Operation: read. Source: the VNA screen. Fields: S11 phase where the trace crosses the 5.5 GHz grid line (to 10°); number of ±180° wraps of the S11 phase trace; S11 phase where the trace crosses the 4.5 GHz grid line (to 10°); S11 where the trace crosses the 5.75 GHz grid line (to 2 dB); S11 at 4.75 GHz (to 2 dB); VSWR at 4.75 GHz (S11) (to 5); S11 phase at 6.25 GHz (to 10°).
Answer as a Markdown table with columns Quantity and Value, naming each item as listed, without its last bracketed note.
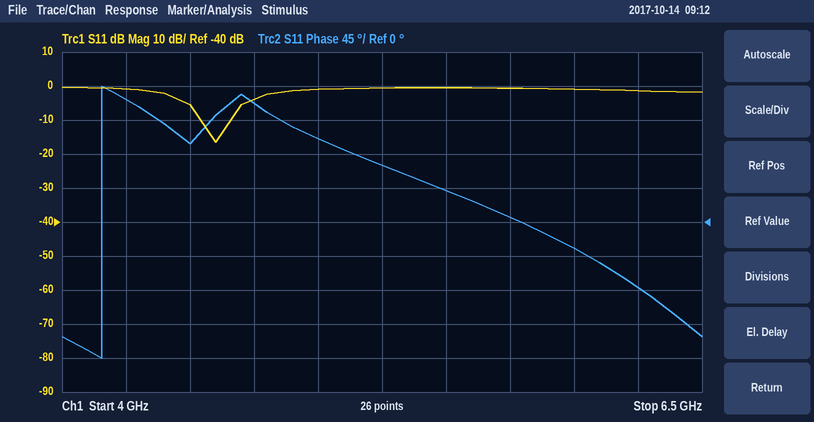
| Quantity | Value |
|---|---|
| S11 phase where the trace crosses the 5.5 GHz grid line | 40° |
| number of ±180° wraps of the S11 phase trace | 1 |
| S11 phase where the trace crosses the 4.5 GHz grid line | 100° |
| S11 where the trace crosses the 5.75 GHz grid line | 0 dB |
| S11 at 4.75 GHz | -4 dB |
| VSWR at 4.75 GHz (S11) | 5 |
| S11 phase at 6.25 GHz | -90° |
